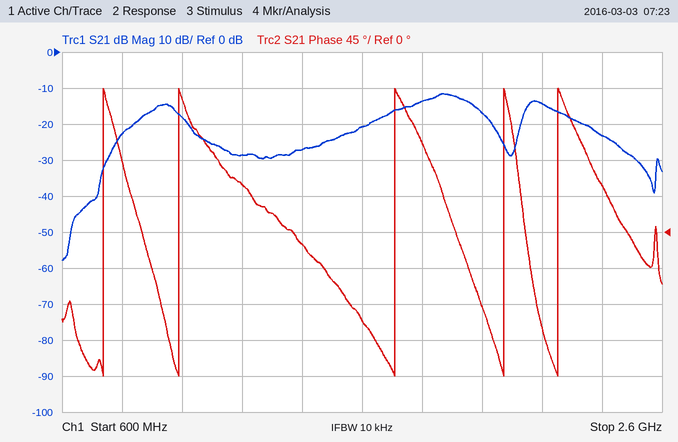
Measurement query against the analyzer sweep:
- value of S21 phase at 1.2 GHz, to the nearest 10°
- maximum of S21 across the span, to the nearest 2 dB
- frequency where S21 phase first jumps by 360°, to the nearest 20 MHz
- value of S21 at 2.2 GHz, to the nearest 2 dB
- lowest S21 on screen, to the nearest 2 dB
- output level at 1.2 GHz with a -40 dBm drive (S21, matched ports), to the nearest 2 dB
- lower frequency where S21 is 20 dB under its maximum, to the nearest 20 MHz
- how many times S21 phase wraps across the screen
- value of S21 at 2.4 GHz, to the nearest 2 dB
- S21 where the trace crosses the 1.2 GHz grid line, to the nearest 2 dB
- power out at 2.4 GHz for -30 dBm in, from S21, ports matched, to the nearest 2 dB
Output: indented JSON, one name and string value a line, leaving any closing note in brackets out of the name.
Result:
{
  "value of S21 phase at 1.2 GHz, to the nearest 10°": "60°",
  "maximum of S21 across the span, to the nearest 2 dB": "-12 dB",
  "frequency where S21 phase first jumps by 360°, to the nearest 20 MHz": "740 MHz",
  "value of S21 at 2.2 GHz, to the nearest 2 dB": "-14 dB",
  "lowest S21 on screen, to the nearest 2 dB": "-58 dB",
  "output level at 1.2 GHz with a -40 dBm drive (S21, matched ports), to the nearest 2 dB": "-68 dBm",
  "lower frequency where S21 is 20 dB under its maximum, to the nearest 20 MHz": "740 MHz",
  "how many times S21 phase wraps across the screen": "5",
  "value of S21 at 2.4 GHz, to the nearest 2 dB": "-24 dB",
  "S21 where the trace crosses the 1.2 GHz grid line, to the nearest 2 dB": "-28 dB",
  "power out at 2.4 GHz for -30 dBm in, from S21, ports matched, to the nearest 2 dB": "-54 dBm"
}
